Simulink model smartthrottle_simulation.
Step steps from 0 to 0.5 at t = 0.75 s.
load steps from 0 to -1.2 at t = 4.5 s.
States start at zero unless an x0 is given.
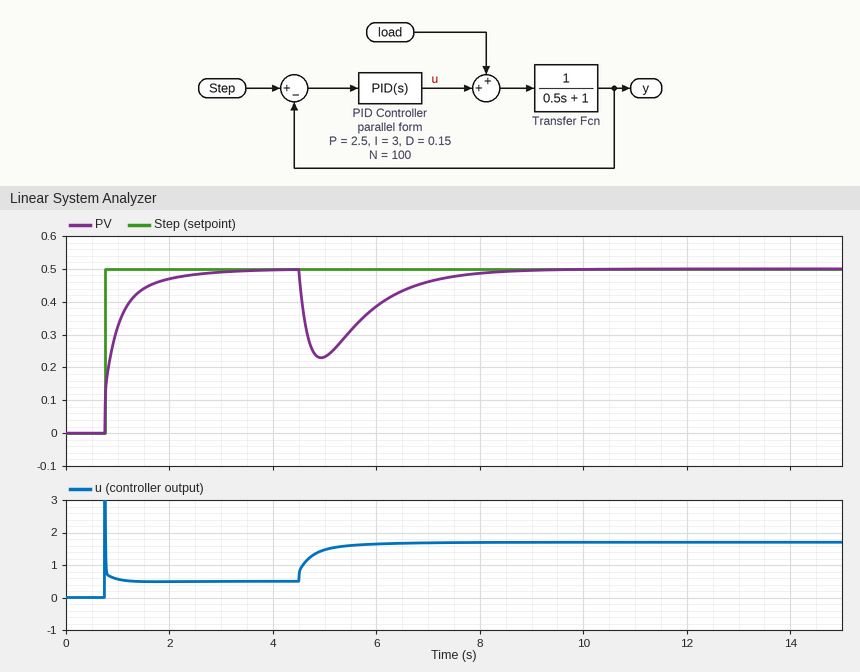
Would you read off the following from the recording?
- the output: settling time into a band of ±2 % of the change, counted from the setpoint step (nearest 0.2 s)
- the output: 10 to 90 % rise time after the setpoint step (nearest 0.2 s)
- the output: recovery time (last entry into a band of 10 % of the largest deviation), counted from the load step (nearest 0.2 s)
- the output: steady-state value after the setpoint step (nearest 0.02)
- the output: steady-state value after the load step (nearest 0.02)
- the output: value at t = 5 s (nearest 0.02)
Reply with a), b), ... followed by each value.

a) 2.2 s
b) 0.8 s
c) 2.8 s
d) 0.50
e) 0.50
f) 0.24
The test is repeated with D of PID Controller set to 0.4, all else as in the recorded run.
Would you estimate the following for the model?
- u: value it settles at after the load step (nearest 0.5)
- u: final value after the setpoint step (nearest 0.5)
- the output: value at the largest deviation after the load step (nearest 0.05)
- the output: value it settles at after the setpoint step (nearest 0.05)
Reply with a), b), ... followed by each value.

a) 1.5
b) 0.5
c) 0.25
d) 0.50
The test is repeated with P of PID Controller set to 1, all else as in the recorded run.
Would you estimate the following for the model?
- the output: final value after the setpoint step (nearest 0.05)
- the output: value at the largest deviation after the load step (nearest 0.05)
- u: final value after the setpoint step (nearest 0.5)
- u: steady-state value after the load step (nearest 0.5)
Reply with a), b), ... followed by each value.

a) 0.50
b) 0.10
c) 0.5
d) 1.5
